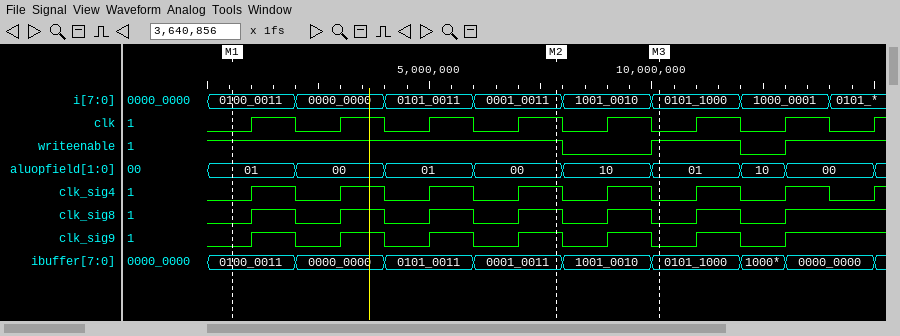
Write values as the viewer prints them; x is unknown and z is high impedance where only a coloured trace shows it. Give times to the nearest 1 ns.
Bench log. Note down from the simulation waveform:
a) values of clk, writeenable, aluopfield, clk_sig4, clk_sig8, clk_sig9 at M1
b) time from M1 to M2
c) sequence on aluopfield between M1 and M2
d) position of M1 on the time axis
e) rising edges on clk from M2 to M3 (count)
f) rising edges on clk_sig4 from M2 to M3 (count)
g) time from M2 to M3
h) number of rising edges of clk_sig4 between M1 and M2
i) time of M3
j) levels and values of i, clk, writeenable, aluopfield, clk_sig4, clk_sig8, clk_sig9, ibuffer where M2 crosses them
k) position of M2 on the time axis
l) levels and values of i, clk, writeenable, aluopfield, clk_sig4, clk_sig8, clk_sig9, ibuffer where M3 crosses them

clk=0, writeenable=1, aluopfield=01, clk_sig4=0, clk_sig8=0, clk_sig9=0
7 ns
01, 00, 01, 00
1 ns
1
1
2 ns
4
10 ns
i=0001_0011, clk=1, writeenable=1, aluopfield=00, clk_sig4=1, clk_sig8=1, clk_sig9=1, ibuffer=0001_0011
8 ns
i=0101_1000, clk=0, writeenable=1, aluopfield=01, clk_sig4=0, clk_sig8=0, clk_sig9=0, ibuffer=0101_1000
